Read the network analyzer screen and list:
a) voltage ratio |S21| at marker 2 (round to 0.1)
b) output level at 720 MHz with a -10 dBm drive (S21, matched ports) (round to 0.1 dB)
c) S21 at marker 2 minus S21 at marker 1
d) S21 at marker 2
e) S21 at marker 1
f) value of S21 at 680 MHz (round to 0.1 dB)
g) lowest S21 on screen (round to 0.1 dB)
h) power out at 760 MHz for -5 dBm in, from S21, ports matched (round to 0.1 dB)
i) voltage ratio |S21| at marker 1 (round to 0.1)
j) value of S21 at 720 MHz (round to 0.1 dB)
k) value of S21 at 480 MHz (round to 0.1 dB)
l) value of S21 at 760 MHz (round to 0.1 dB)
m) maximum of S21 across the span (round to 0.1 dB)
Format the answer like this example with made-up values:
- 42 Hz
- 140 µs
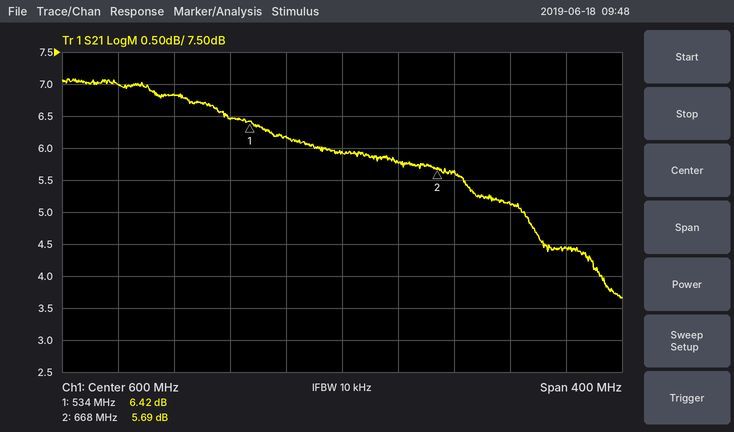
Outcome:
- 1.9
- -4.9 dBm
- -0.73 dB
- 5.69 dB
- 6.42 dB
- 5.6 dB
- 3.7 dB
- -0.6 dBm
- 2.1
- 5.1 dB
- 6.8 dB
- 4.4 dB
- 7.1 dB
